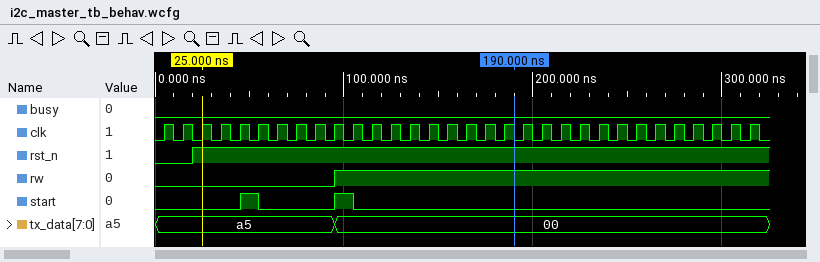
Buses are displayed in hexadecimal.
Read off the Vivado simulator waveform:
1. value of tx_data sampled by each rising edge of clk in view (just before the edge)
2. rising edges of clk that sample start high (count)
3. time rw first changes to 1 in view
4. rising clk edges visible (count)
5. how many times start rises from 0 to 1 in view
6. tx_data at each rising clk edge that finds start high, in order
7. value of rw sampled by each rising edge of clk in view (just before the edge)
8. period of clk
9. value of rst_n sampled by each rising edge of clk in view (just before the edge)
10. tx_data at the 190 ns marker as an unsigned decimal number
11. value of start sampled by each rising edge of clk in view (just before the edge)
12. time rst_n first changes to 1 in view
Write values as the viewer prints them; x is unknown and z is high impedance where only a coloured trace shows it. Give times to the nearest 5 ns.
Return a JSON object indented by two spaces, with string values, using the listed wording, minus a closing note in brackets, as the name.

{
  "value of tx_data sampled by each rising edge of clk in view": "a5, a5, a5, a5, a5, a5, a5, a5, a5, a5, 00, 00, 00, 00, 00, 00, 00, 00, 00, 00, 00, 00, 00, 00, 00, 00, 00, 00, 00, 00, 00, 00",
  "rising edges of clk that sample start high": "2",
  "time rw first changes to 1 in view": "95 ns",
  "rising clk edges visible": "32",
  "how many times start rises from 0 to 1 in view": "2",
  "tx_data at each rising clk edge that finds start high, in order": "a5, 00",
  "value of rw sampled by each rising edge of clk in view": "0 0 0 0 0 0 0 0 0 0 1 1 1 1 1 1 1 1 1 1 1 1 1 1 1 1 1 1 1 1 1 1",
  "period of clk": "10 ns",
  "value of rst_n sampled by each rising edge of clk in view": "0 0 1 1 1 1 1 1 1 1 1 1 1 1 1 1 1 1 1 1 1 1 1 1 1 1 1 1 1 1 1 1",
  "tx_data at the 190 ns marker as an unsigned decimal number": "0",
  "value of start sampled by each rising edge of clk in view": "0 0 0 0 0 1 0 0 0 0 1 0 0 0 0 0 0 0 0 0 0 0 0 0 0 0 0 0 0 0 0 0",
  "time rst_n first changes to 1 in view": "20 ns"
}
